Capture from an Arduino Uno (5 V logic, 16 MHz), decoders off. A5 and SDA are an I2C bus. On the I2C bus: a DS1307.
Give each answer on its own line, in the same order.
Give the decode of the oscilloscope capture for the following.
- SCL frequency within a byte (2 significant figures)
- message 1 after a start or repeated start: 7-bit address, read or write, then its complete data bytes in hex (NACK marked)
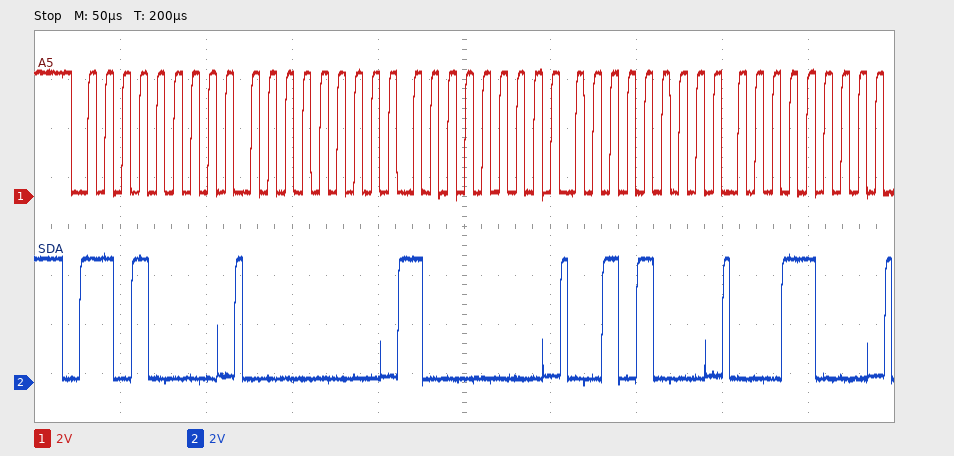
100 kHz
0x68 write: 00 80 28 18
